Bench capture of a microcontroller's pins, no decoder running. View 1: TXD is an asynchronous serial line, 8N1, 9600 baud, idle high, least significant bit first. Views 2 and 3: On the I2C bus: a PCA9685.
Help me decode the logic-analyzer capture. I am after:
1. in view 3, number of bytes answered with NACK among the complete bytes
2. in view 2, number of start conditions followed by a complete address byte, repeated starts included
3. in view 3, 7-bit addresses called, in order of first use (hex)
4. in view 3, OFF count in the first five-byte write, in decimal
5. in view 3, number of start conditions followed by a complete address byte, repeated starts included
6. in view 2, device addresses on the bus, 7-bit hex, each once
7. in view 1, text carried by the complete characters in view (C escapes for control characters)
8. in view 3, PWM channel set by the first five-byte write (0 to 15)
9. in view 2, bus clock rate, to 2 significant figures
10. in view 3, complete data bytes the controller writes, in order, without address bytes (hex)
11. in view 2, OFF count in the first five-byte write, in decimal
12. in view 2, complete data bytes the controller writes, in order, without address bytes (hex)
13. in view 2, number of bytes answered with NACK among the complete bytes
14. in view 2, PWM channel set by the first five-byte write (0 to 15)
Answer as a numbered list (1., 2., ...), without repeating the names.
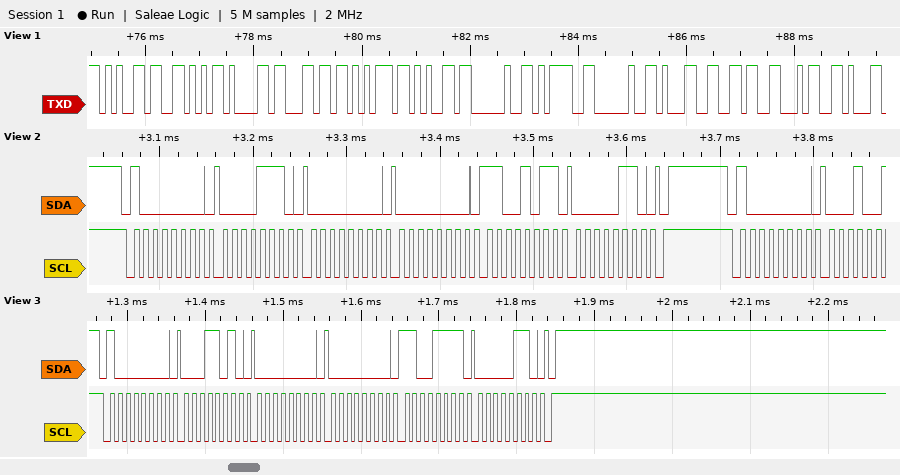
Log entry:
1. 0
2. 2
3. 0x40
4. 1743
5. 1
6. 0x40
7. "eValue = 164"
8. 5
9. 100 kHz
10. 1A 00 00 CF 06
11. 1739
12. 0E 00 00 CB 06
13. 0
14. 2
